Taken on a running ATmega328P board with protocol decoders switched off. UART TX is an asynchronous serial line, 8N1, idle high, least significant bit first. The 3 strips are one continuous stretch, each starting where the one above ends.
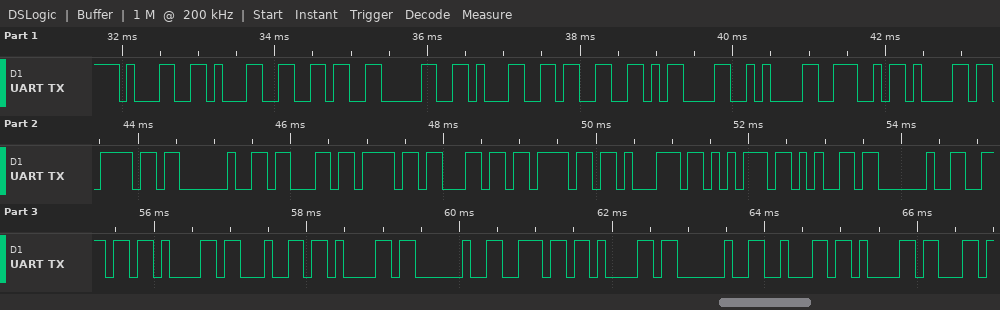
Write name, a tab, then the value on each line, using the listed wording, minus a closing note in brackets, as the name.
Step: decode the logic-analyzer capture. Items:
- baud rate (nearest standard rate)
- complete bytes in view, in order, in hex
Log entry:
baud rate	9600 baud
complete bytes in view, in order, in hex	31 31 36 30 31 33 0D 0A 4E 61 6F 20 63 6F 6C 6F 71 75 65 20 6E 61 64 61 20 6E 61 20 62 61
